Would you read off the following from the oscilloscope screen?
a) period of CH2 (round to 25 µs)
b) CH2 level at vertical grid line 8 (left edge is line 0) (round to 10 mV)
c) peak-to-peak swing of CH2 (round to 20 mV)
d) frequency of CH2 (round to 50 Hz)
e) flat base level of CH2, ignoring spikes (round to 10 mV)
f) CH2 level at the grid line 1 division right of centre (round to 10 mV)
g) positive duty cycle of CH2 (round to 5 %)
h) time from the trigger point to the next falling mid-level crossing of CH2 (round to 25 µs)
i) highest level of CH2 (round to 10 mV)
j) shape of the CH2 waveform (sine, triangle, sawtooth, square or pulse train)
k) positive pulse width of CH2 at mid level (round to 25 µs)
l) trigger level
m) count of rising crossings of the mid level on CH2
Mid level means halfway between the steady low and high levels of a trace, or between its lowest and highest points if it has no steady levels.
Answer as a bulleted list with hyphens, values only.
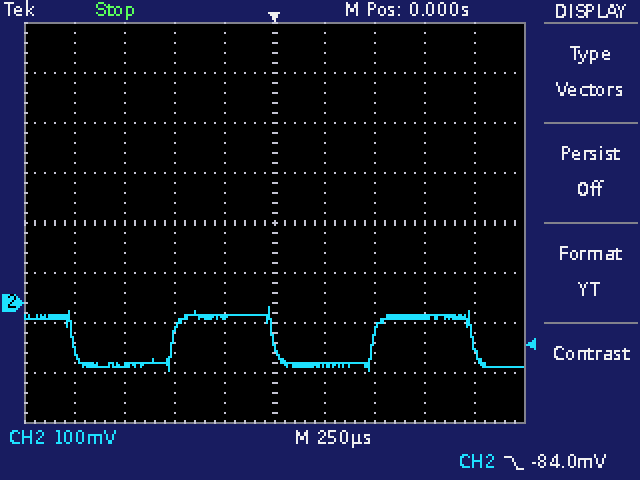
- 1.000 ms
- -30 mV
- 120 mV
- 1.00 kHz
- -120 mV
- -120 mV
- 50 %
- 1.000 ms
- -10 mV
- square
- 500 µs
- -84.0 mV
- 2
